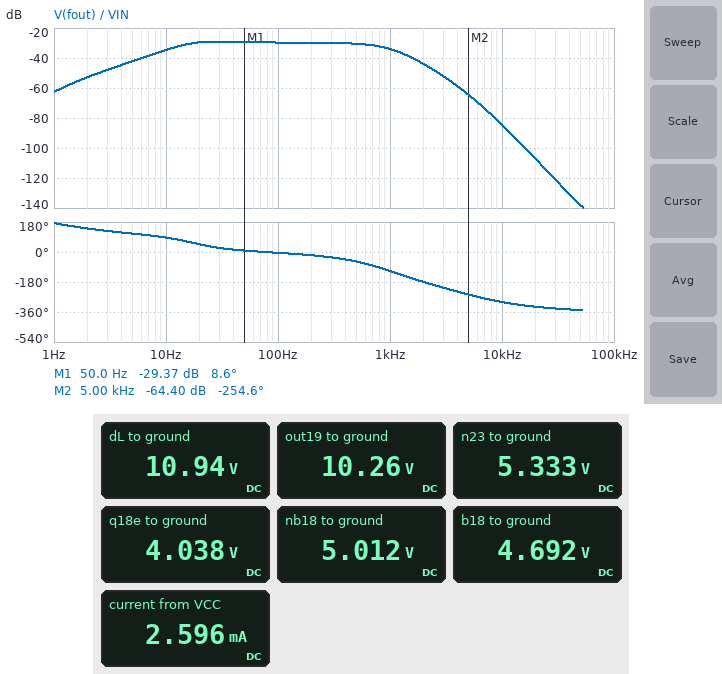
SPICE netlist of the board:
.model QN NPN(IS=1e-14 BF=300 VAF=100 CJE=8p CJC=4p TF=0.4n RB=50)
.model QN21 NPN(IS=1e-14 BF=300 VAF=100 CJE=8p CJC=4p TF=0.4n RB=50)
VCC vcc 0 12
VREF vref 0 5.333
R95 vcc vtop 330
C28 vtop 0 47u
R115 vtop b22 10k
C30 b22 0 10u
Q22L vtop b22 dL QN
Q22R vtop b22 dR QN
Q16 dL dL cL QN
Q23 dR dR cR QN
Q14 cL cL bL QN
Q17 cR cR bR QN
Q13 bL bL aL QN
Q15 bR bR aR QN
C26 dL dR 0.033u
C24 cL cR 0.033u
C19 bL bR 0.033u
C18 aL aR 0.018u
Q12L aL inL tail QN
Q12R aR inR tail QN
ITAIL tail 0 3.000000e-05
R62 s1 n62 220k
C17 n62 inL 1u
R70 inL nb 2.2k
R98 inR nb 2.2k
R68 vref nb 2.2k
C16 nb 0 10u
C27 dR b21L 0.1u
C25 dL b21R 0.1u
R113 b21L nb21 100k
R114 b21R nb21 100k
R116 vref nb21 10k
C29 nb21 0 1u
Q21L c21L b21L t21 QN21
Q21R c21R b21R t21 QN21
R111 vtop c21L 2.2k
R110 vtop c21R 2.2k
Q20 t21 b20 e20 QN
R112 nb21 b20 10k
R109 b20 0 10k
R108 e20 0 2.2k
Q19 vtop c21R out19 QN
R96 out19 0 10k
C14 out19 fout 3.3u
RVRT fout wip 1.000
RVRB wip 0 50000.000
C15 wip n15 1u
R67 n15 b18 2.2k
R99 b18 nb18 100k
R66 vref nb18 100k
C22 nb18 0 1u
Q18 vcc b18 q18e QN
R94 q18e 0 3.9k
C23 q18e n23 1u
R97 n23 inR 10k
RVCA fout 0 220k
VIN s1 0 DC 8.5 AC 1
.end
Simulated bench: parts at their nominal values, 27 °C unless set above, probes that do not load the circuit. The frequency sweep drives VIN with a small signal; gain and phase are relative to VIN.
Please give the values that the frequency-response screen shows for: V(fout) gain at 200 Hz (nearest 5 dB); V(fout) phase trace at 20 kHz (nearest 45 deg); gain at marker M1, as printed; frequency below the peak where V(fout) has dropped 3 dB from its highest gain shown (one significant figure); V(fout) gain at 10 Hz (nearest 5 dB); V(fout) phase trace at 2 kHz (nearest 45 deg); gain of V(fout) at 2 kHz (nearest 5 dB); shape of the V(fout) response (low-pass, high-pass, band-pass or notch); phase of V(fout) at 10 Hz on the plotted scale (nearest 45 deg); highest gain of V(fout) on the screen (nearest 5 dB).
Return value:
-30 dB
-315 deg
-29.37 dB
10 Hz
-35 dB
-180 deg
-45 dB
band-pass
90 deg
-30 dB
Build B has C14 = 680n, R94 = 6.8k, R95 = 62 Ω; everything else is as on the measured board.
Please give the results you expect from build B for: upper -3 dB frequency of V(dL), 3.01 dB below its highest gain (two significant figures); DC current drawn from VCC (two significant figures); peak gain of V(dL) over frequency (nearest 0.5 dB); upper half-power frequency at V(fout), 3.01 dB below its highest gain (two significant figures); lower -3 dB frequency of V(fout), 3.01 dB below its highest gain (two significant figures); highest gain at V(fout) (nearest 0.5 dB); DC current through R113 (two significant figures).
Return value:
29 Hz
2.2 mA
-44.0 dB
690 Hz
15 Hz
-28.5 dB
780 nA
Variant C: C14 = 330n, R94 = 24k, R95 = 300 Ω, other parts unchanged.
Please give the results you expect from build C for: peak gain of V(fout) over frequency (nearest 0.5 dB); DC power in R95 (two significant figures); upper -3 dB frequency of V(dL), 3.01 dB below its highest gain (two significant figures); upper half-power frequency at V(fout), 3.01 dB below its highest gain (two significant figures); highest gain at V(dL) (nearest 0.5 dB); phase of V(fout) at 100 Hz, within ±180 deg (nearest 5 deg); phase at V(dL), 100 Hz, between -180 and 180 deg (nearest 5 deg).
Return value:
-28.0 dB
740 µW
32 Hz
610 Hz
-43.5 dB
0 deg
135 deg
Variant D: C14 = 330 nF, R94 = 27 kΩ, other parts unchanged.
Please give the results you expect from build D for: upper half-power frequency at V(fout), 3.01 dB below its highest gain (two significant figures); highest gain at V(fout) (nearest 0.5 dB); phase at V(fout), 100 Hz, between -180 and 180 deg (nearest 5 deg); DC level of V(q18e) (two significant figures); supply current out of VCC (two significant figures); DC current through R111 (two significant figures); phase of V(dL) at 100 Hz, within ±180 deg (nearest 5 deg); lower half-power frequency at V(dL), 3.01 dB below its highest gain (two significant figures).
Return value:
610 Hz
-28.0 dB
0 deg
4.6 V
1.7 mA
250 µA
135 deg
1.9 Hz
